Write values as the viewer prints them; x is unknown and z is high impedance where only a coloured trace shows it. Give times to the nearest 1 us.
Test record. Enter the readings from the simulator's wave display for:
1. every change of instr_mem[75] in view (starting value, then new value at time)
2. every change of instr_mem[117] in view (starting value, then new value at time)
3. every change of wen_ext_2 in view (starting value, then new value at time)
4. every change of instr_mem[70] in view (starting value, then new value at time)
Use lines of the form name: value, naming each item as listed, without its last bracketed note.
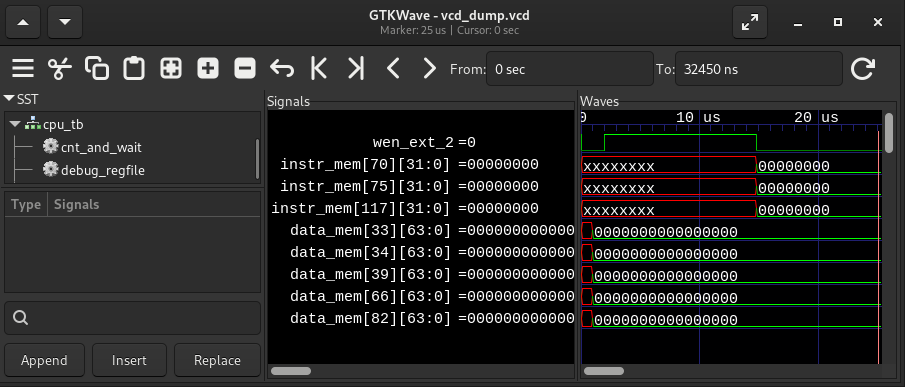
every change of instr_mem[75] in view: xxxxxxxx, 00000000 at 15 us
every change of instr_mem[117] in view: xxxxxxxx, 00000000 at 15 us
every change of wen_ext_2 in view: 0, 1 at 2 us, 0 at 15 us
every change of instr_mem[70] in view: xxxxxxxx, 00000000 at 15 us
